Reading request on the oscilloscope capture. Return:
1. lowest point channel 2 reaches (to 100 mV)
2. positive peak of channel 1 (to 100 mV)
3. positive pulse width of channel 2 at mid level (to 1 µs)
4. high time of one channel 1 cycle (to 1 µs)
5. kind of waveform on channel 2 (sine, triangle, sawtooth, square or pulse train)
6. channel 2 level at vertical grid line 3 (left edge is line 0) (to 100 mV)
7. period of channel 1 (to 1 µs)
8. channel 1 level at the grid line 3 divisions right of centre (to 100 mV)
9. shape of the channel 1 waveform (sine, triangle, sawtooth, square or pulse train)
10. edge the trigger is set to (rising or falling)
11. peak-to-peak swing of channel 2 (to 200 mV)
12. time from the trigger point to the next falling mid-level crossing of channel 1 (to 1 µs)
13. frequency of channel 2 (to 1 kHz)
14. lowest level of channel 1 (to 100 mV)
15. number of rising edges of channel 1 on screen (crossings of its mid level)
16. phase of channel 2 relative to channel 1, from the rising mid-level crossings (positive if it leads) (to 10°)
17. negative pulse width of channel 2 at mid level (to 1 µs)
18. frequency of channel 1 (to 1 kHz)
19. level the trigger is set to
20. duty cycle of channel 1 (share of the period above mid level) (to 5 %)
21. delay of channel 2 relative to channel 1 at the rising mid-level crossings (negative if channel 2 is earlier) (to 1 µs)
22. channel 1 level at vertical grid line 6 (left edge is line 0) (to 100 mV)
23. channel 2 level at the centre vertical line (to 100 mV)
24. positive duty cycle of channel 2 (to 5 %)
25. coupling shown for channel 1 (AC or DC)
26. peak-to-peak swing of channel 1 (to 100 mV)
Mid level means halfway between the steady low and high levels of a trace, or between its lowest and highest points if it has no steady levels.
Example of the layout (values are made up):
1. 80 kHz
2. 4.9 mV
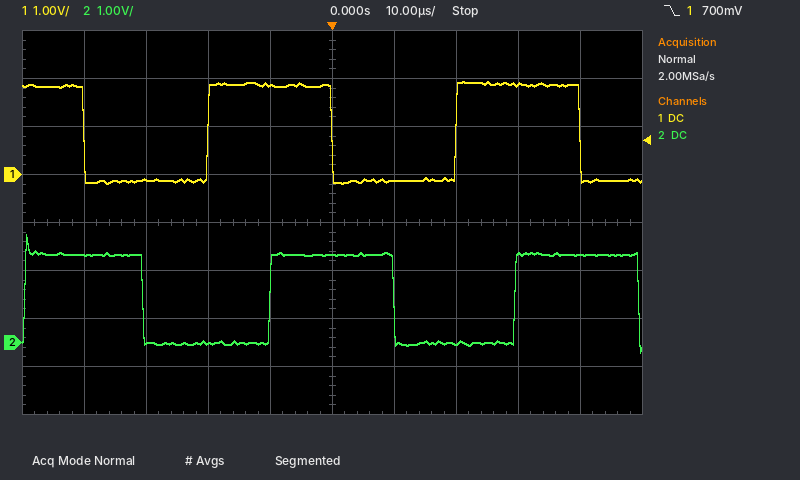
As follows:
1. -200 mV
2. 1.9 V
3. 20 µs
4. 20 µs
5. square
6. 0.0 V
7. 40 µs
8. 1.9 V
9. square
10. falling
11. 2.4 V
12. 40 µs
13. 25 kHz
14. -200 mV
15. 2
16. -90°
17. 20 µs
18. 25 kHz
19. 700 mV
20. 50 %
21. +10 µs
22. -100 mV
23. 1.8 V
24. 50 %
25. DC
26. 2.1 V
